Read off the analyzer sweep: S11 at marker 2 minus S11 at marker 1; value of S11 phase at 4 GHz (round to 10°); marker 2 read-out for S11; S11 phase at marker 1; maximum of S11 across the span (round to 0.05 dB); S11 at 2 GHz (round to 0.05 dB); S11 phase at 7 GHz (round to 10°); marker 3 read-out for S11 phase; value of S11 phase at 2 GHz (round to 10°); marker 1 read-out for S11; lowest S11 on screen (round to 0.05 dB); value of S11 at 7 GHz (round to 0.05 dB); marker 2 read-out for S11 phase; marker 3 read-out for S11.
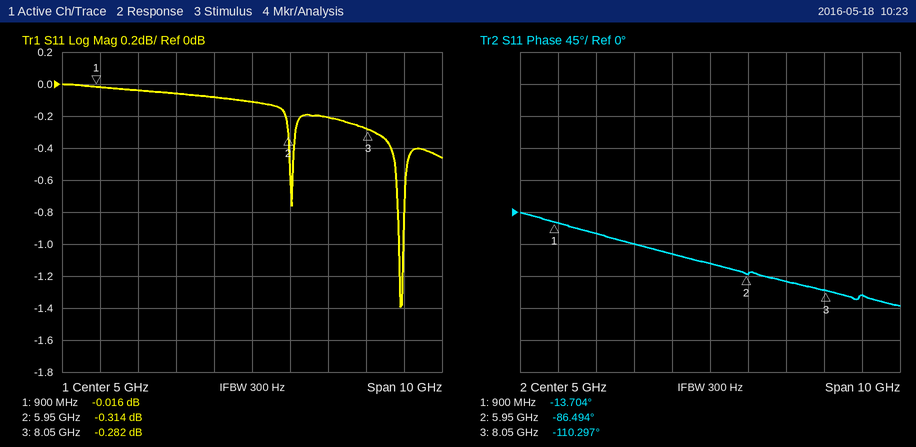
-0.298 dB
-60°
-0.314 dB
-13.704°
0.00 dB
-0.05 dB
-100°
-110.297°
-30°
-0.016 dB
-1.40 dB
-0.20 dB
-86.494°
-0.282 dB
